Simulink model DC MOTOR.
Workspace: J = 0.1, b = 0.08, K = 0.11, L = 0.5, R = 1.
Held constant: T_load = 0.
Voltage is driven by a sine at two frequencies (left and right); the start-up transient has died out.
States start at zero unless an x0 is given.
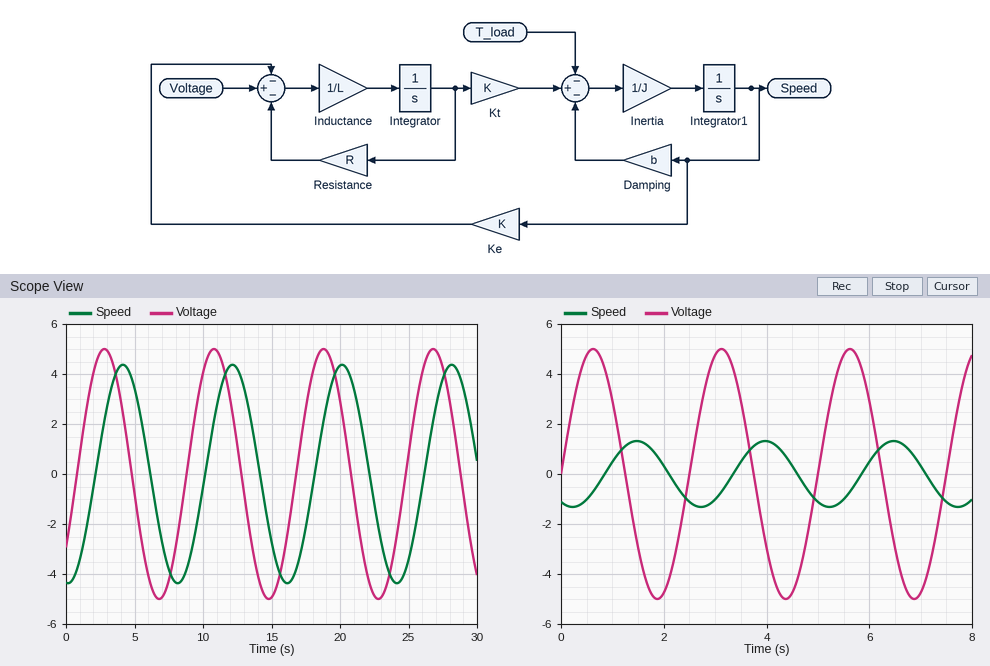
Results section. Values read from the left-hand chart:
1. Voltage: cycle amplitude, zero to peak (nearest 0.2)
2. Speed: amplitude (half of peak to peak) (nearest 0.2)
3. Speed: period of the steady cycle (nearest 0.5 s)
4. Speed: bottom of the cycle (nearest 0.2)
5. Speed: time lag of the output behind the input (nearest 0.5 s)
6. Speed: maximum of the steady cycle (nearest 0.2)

5.0
4.4
8.0 s
-4.4
1.5 s
4.4
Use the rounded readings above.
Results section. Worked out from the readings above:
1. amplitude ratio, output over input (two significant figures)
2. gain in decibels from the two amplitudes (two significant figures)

0.88
-1.1 dB
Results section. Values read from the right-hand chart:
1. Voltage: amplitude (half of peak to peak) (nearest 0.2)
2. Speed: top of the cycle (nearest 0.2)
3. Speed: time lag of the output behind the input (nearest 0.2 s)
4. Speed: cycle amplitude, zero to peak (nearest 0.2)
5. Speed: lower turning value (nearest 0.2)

5.0
1.4
0.8 s
1.4
-1.4
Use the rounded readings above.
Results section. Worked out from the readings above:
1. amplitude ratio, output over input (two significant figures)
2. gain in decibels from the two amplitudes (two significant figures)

0.28
-11 dB
